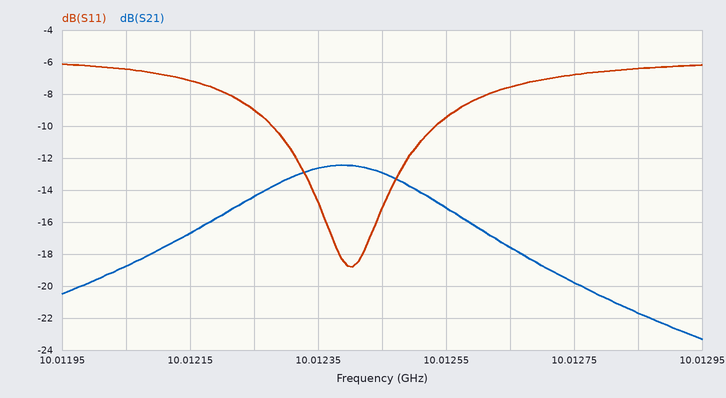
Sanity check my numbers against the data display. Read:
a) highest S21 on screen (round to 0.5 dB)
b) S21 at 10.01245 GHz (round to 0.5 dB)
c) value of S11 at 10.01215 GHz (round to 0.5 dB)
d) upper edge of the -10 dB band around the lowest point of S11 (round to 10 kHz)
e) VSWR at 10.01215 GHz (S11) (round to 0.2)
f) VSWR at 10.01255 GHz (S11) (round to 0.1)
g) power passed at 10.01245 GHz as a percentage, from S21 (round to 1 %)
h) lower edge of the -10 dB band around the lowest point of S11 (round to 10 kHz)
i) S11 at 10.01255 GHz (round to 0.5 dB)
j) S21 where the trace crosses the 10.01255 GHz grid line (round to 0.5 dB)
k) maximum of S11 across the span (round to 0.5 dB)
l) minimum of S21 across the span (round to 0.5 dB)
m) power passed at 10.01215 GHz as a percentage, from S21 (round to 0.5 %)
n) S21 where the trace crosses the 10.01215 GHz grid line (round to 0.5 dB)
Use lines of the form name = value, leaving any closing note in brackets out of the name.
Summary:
highest S21 on screen = -12.5 dB
S21 at 10.01245 GHz = -13.0 dB
value of S11 at 10.01215 GHz = -7.0 dB
upper edge of the -10 dB band around the lowest point of S11 = 10.01253 GHz
VSWR at 10.01215 GHz (S11) = 2.6
VSWR at 10.01255 GHz (S11) = 2.0
power passed at 10.01245 GHz as a percentage, from S21 = 5 %
lower edge of the -10 dB band around the lowest point of S11 = 10.01228 GHz
S11 at 10.01255 GHz = -9.5 dB
S21 where the trace crosses the 10.01255 GHz grid line = -15.0 dB
maximum of S11 across the span = -6.0 dB
minimum of S21 across the span = -23.5 dB
power passed at 10.01215 GHz as a percentage, from S21 = 2.0 %
S21 where the trace crosses the 10.01215 GHz grid line = -16.5 dB
